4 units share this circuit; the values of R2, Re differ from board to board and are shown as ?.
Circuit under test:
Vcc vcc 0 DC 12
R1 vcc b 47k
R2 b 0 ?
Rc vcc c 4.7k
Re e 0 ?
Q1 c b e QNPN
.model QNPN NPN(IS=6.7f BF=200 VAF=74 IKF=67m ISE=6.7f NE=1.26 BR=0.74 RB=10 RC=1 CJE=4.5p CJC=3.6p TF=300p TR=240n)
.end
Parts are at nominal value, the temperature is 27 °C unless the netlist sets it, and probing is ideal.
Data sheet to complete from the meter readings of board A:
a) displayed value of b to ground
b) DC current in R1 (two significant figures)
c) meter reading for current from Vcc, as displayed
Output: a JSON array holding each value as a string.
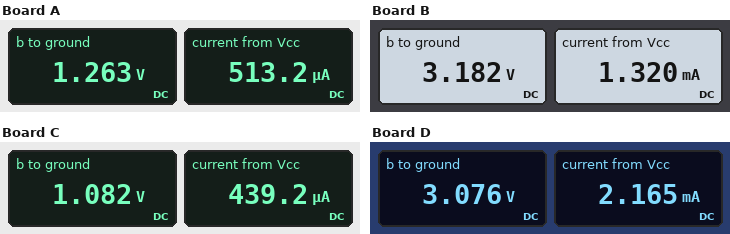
["1.263 V", "230 µA", "513.2 µA"]
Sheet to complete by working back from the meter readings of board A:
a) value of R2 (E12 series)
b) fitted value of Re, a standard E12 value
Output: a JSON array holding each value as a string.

["5.6 kΩ", "2.2 kΩ"]
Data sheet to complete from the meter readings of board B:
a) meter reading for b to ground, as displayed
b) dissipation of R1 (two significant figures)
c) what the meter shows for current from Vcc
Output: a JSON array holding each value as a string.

["3.182 V", "1.7 mW", "1.320 mA"]
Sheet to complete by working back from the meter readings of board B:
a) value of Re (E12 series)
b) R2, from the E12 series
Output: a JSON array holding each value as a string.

["2.2 kΩ", "18 kΩ"]
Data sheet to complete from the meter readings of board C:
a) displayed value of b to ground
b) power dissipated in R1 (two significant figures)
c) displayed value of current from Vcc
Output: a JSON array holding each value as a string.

["1.082 V", "2.5 mW", "439.2 µA"]
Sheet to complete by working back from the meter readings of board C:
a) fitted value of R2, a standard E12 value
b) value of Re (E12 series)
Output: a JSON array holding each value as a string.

["4.7 kΩ", "2.2 kΩ"]
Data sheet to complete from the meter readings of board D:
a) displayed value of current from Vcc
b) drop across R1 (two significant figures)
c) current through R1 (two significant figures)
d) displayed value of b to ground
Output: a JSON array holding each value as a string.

["2.165 mA", "8.9 V", "190 µA", "3.076 V"]
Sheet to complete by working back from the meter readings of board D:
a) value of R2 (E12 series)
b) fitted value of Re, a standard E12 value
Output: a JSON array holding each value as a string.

["18 kΩ", "1.2 kΩ"]
